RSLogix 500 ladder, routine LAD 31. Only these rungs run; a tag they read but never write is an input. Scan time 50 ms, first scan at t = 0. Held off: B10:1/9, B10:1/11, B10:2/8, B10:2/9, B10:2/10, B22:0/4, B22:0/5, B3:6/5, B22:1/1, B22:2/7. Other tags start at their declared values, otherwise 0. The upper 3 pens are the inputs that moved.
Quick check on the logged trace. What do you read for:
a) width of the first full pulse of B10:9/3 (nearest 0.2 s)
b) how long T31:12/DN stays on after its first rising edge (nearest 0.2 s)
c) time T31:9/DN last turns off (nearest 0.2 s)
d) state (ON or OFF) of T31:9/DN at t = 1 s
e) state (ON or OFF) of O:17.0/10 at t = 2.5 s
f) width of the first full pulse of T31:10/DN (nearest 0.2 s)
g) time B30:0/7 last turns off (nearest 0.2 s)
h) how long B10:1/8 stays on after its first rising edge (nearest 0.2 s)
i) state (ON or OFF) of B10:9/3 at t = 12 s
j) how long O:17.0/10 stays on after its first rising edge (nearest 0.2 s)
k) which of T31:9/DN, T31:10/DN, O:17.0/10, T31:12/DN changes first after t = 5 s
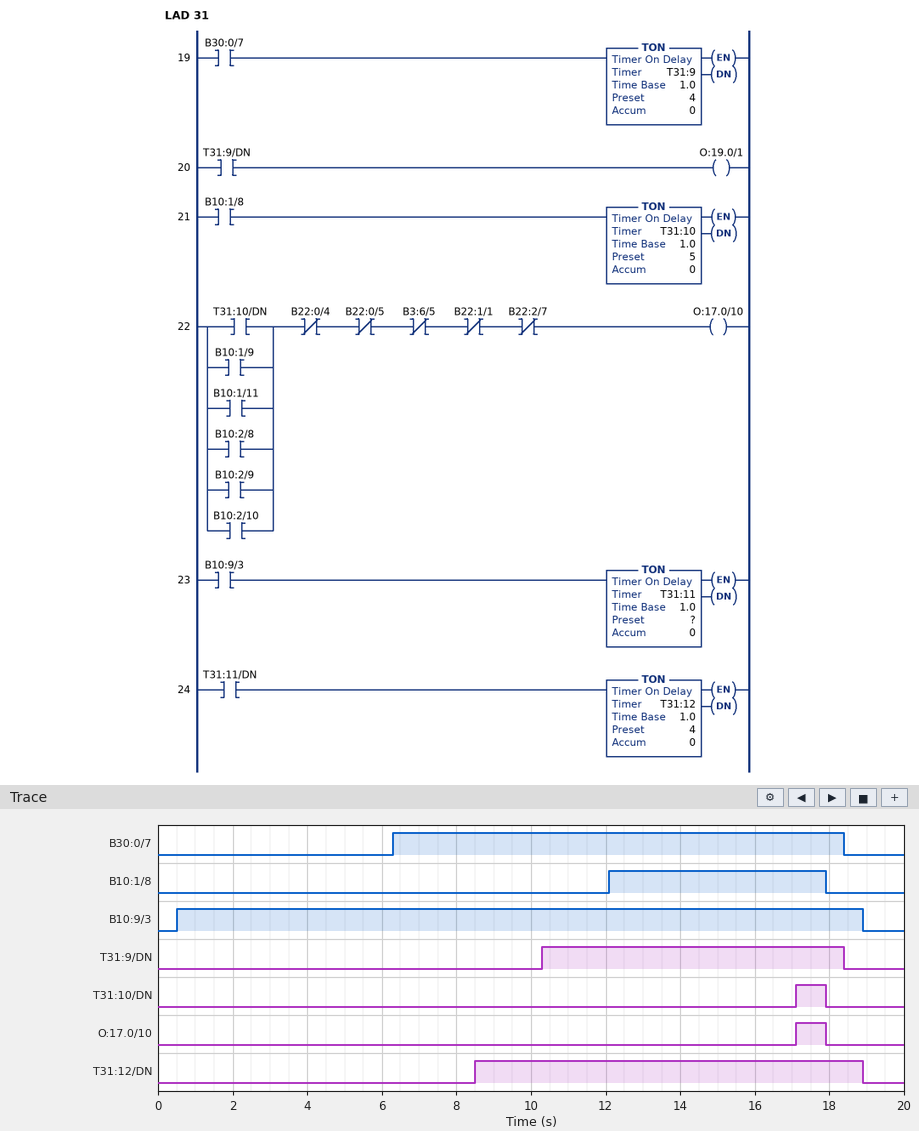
18.4 s
10.4 s
18.4 s
OFF
OFF
0.8 s
18.4 s
5.8 s
ON
0.8 s
T31:12/DN
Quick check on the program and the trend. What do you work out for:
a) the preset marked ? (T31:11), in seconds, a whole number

4 s
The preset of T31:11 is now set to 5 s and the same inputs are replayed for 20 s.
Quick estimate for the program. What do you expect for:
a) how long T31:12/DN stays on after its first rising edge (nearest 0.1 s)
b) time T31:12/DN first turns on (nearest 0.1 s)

9.4 s
9.5 s
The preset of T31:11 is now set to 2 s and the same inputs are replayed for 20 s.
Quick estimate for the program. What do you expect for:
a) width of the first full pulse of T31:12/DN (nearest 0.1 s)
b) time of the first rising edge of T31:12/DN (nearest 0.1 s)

12.4 s
6.5 s
